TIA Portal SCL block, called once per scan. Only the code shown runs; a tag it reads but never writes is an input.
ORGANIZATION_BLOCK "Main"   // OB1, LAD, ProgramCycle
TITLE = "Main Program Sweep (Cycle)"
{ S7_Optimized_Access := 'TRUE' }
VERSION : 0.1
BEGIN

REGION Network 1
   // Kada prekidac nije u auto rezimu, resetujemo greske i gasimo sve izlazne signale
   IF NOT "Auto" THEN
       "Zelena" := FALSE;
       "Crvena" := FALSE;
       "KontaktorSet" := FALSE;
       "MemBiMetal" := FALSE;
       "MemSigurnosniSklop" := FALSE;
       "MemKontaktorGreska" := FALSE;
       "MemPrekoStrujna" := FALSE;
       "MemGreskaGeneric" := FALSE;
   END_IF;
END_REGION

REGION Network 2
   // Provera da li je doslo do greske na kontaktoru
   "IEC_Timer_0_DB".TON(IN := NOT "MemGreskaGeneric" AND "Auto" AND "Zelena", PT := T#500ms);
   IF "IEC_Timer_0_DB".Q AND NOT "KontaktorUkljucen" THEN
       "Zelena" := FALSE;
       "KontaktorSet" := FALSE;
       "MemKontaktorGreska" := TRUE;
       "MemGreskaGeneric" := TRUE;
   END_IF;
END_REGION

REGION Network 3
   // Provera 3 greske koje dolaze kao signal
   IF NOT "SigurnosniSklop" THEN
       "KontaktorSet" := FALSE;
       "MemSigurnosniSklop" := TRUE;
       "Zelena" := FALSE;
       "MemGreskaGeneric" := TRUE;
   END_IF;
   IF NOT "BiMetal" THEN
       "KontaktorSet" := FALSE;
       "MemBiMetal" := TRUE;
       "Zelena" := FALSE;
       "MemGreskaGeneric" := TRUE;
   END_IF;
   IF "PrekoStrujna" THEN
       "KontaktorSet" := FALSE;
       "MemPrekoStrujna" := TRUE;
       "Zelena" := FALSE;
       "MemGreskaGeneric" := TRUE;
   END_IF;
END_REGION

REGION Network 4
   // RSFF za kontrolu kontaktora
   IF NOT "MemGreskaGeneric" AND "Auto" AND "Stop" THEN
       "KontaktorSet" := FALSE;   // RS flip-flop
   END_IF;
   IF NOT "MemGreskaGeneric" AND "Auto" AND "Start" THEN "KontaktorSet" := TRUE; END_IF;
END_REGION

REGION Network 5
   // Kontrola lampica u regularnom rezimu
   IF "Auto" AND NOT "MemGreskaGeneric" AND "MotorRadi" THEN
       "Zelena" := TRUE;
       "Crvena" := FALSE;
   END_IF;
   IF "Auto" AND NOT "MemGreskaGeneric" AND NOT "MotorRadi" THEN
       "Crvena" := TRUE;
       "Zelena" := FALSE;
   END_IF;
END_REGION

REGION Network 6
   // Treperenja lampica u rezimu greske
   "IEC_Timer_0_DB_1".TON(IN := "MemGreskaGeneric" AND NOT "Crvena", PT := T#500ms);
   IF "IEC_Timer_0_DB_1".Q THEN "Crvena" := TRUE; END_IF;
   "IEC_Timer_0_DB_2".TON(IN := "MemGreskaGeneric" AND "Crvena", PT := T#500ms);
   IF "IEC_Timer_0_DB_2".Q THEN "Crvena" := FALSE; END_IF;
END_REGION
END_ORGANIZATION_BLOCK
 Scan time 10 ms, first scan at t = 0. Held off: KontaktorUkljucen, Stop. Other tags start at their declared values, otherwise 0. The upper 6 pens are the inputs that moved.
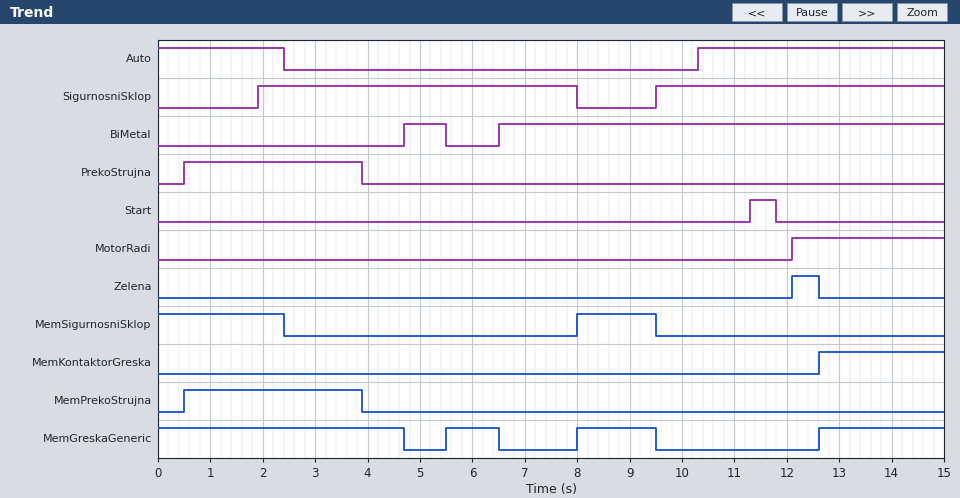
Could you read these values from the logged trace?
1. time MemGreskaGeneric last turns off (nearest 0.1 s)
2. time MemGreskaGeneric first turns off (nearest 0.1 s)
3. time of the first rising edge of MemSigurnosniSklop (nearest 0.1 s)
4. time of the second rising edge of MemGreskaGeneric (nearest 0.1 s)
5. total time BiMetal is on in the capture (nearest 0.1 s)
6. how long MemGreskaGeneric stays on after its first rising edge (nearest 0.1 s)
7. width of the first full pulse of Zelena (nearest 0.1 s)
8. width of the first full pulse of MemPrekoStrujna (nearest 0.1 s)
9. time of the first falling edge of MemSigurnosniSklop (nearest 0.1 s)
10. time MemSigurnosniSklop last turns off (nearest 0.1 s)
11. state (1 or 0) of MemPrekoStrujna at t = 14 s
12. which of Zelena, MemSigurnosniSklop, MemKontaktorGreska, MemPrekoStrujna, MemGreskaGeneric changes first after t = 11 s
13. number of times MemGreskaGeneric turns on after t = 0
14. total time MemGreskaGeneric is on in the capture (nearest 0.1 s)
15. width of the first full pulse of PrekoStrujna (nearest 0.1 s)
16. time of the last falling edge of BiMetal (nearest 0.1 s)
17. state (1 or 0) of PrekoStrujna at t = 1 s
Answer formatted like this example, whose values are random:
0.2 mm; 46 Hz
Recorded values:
9.5 s; 4.7 s; 8.0 s; 8.0 s; 9.3 s; 1.0 s; 0.5 s; 3.4 s; 2.4 s; 9.5 s; 0; Zelena; 3; 9.6 s; 3.4 s; 5.5 s; 1
